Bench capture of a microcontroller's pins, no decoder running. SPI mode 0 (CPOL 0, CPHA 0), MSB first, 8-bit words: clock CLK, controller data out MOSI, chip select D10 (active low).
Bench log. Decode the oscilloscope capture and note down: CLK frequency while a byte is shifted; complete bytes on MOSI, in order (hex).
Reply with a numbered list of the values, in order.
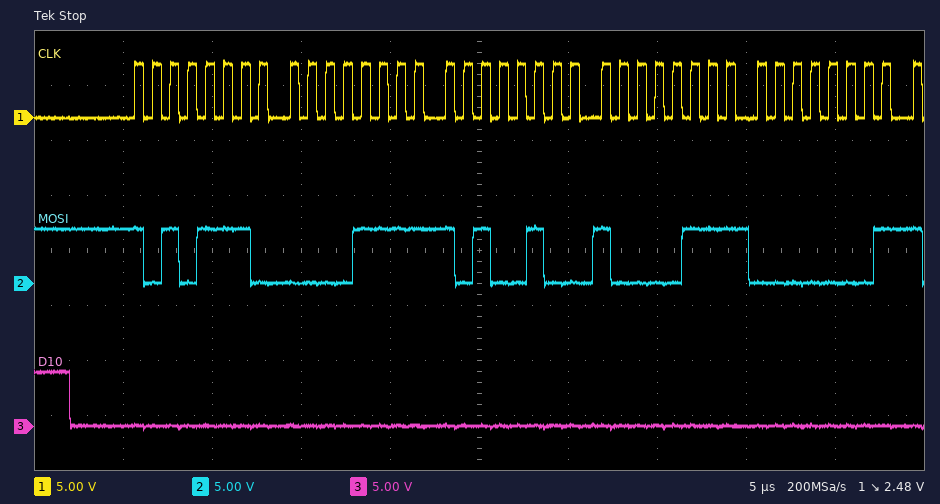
1. 1 MHz
2. AE 0F A4 87 01
